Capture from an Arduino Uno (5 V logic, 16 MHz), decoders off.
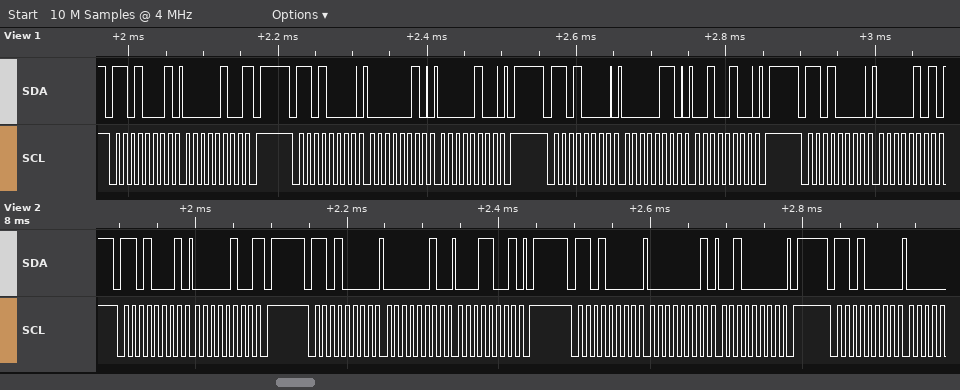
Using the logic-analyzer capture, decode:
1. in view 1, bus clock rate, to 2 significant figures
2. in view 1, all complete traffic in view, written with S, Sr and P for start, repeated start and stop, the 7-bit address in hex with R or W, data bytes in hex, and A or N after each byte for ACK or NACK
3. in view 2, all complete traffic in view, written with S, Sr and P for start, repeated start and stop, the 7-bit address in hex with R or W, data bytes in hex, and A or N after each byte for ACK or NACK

100 kHz
S 68R A 04 N P S 68W A 02 A 04 A P S 68W A 06 A 24 A P S 68W A 05 A
S 68R A 04 N P S 68W A 02 A 19 A P S 68W A 01 A 20 A P S 68W A
